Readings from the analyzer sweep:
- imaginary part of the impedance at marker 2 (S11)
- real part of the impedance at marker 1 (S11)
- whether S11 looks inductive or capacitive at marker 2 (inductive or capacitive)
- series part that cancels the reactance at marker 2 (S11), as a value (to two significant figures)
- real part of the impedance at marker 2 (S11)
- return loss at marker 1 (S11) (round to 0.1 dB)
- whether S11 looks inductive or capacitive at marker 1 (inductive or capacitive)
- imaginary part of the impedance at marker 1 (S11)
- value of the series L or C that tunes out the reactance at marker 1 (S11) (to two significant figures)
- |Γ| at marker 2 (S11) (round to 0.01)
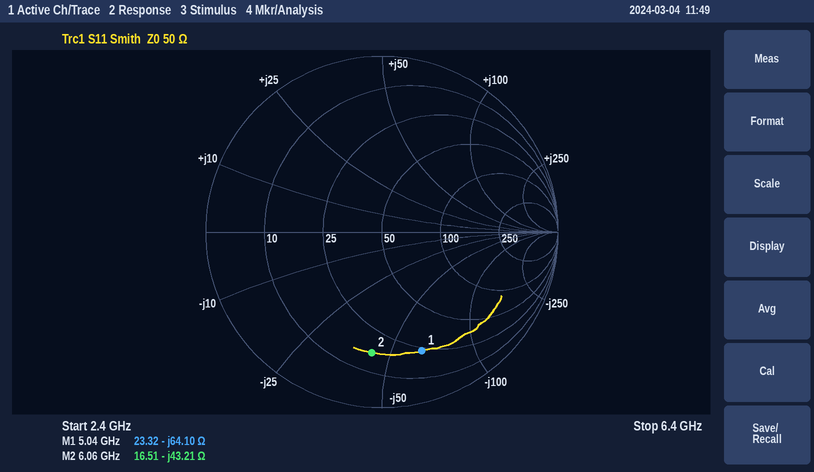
-43.21 Ω
23.32 Ω
capacitive
1.1 nH
16.51 Ω
2.9 dB
capacitive
-64.10 Ω
2.0 nH
0.69
